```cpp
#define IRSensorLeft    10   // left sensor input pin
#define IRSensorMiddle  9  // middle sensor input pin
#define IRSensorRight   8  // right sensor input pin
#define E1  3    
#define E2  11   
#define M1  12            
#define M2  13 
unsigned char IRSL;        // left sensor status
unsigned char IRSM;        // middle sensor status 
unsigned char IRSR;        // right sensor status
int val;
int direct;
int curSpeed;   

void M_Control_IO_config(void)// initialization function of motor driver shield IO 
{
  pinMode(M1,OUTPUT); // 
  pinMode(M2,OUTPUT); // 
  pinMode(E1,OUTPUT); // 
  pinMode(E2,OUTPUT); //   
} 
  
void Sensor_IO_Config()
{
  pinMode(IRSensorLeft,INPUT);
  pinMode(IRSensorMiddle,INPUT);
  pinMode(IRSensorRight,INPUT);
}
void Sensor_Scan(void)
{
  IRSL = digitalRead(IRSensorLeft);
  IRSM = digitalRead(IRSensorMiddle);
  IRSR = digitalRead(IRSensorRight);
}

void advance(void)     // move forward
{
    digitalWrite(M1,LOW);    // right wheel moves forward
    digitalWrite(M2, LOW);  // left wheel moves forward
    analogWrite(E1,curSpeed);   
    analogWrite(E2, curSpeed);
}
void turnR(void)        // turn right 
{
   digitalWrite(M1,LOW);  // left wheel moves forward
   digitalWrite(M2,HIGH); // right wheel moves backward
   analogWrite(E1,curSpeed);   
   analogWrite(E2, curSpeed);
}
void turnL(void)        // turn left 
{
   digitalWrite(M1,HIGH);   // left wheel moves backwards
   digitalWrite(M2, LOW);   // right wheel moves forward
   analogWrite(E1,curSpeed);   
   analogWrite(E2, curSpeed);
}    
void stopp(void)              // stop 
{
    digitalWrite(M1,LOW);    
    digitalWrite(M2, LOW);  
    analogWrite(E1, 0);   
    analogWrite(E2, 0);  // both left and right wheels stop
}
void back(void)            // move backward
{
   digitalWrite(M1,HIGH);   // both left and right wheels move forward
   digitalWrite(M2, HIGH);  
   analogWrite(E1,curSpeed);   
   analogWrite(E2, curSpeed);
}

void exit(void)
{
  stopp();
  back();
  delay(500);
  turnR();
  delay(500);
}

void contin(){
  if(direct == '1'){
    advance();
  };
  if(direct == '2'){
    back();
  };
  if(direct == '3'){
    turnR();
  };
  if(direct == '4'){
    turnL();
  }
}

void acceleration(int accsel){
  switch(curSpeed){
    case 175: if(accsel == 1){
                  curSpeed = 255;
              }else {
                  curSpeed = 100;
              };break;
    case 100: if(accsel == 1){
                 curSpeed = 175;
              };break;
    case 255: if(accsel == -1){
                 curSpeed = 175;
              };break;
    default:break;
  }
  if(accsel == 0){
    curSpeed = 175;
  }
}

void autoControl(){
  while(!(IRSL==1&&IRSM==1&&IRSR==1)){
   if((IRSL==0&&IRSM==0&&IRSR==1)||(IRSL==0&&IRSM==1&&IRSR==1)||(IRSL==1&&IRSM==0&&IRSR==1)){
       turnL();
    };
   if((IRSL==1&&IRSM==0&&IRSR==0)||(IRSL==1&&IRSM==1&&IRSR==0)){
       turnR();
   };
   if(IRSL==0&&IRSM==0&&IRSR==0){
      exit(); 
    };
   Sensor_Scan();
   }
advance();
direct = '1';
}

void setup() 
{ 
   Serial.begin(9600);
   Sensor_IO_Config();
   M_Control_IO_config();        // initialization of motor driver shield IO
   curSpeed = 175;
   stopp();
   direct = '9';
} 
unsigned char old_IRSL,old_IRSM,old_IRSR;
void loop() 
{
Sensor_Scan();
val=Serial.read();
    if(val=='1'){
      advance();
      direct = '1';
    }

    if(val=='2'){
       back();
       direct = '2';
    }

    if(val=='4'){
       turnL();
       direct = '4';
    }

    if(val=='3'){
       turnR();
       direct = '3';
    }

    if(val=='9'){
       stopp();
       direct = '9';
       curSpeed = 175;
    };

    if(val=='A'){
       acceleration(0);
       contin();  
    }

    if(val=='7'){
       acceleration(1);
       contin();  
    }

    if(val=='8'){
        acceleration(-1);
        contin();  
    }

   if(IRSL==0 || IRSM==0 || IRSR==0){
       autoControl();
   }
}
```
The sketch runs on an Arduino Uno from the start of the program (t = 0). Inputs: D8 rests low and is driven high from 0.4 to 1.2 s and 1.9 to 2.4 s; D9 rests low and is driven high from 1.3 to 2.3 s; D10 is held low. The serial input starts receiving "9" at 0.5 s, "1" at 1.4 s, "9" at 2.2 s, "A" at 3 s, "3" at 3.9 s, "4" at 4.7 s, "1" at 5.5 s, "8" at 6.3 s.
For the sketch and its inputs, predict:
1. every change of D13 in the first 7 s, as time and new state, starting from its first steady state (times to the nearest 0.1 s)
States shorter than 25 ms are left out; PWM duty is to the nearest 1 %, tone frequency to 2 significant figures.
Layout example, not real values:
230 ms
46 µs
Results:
0 s high; 1 s low; 1.2 s high; 2.2 s low; 2.4 s high
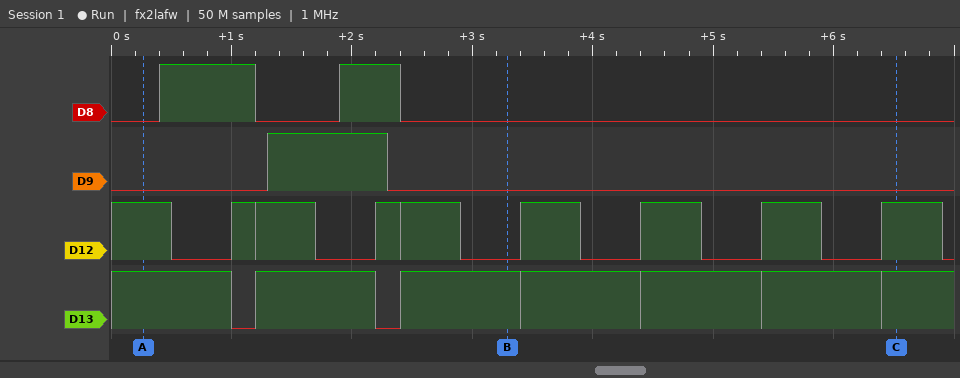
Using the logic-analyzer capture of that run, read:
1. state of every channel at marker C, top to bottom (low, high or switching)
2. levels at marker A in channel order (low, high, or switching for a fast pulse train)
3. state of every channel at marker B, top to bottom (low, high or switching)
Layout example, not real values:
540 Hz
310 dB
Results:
D8 low, D9 low, D12 high, D13 high
D8 low, D9 low, D12 high, D13 high
D8 low, D9 low, D12 low, D13 high
